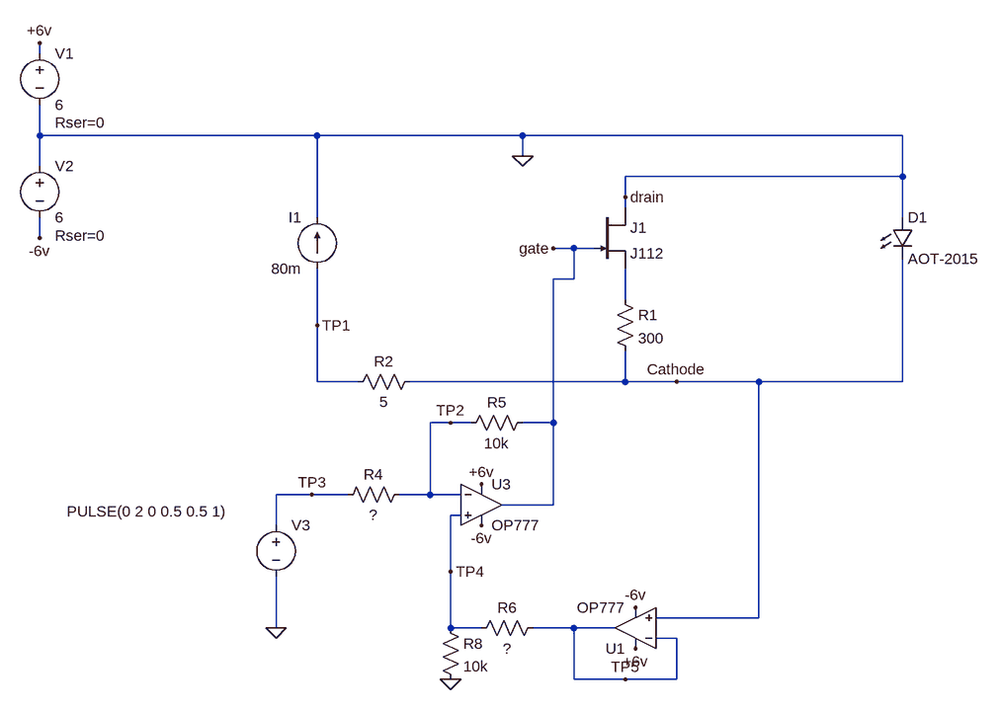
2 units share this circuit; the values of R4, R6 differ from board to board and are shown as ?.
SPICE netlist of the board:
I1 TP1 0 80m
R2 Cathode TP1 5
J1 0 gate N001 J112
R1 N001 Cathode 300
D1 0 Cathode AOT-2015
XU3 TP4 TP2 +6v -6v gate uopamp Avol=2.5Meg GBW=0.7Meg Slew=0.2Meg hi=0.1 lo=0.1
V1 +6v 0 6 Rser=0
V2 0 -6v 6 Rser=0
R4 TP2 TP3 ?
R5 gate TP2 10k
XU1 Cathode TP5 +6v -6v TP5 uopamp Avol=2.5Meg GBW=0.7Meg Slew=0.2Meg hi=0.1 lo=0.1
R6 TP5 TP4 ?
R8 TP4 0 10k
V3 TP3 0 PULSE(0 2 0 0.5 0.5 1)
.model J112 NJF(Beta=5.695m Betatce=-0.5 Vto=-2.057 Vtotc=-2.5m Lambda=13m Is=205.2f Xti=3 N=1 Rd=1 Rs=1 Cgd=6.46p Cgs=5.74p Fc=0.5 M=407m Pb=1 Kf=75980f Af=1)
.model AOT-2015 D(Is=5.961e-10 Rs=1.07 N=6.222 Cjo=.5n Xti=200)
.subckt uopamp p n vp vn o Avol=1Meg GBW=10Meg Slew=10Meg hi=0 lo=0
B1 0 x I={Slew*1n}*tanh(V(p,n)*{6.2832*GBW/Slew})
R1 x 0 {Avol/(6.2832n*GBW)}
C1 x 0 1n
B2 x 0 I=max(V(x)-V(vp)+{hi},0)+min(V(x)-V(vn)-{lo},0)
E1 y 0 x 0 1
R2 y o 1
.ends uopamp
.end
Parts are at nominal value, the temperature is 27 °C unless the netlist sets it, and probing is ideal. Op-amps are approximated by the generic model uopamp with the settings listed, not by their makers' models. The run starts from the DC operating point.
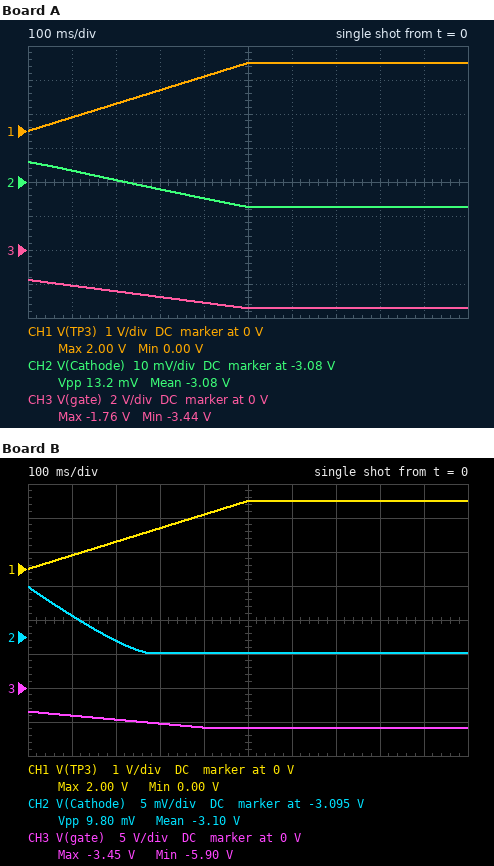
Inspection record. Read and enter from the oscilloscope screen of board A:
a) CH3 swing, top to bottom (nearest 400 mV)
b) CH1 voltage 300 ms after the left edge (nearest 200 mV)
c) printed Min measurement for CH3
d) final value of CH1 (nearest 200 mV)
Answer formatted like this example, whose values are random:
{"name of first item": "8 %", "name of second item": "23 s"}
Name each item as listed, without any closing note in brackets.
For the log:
{"CH3 swing, top to bottom": "1.6 V", "CH1 voltage 300 ms after the left edge": "1.2 V", "printed Min measurement for CH3": "-3.44 V", "final value of CH1": "2.0 V"}
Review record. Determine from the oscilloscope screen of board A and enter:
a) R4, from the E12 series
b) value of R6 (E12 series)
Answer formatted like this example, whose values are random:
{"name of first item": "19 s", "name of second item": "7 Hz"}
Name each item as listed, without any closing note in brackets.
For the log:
{"R4, from the E12 series": "12 kΩ", "value of R6": "22 kΩ"}
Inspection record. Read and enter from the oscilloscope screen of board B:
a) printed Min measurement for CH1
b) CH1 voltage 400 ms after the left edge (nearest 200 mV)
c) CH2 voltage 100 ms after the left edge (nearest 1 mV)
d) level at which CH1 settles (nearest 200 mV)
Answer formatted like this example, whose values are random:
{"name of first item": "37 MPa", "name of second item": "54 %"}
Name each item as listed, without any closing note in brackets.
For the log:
{"printed Min measurement for CH1": "0.00 V", "CH1 voltage 400 ms after the left edge": "1.6 V", "CH2 voltage 100 ms after the left edge": "-3.092 V", "level at which CH1 settles": "2.0 V"}
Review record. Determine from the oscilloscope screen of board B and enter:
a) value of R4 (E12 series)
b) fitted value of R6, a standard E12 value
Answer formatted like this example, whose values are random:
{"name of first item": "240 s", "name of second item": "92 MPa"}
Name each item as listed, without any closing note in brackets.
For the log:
{"value of R4": "6.8 kΩ", "fitted value of R6, a standard E12 value": "12 kΩ"}
